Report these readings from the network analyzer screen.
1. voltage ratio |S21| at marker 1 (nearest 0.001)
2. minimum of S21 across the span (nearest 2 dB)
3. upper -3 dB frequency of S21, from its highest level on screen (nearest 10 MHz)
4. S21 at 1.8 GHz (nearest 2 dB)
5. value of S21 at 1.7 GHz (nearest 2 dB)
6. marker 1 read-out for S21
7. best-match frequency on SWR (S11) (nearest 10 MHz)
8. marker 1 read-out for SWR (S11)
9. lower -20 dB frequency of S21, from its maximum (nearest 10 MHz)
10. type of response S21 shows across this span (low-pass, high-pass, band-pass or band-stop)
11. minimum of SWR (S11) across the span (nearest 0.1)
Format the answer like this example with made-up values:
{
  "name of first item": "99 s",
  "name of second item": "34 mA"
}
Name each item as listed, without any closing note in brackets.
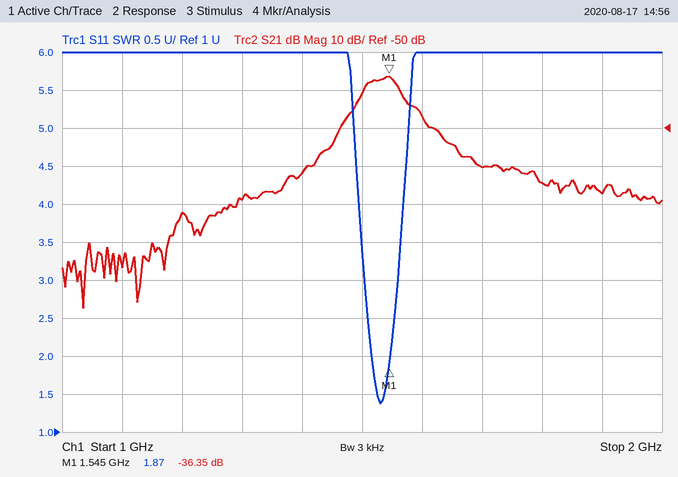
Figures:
{
  "voltage ratio |S21| at marker 1": "0.015",
  "minimum of S21 across the span": "-98 dB",
  "upper -3 dB frequency of S21, from its highest level on screen": "1.56 GHz",
  "S21 at 1.8 GHz": "-64 dB",
  "value of S21 at 1.7 GHz": "-60 dB",
  "marker 1 read-out for S21": "-36.35 dB",
  "best-match frequency on SWR (S11)": "1.53 GHz",
  "marker 1 read-out for SWR": "1.87",
  "lower -20 dB frequency of S21, from its maximum": "1.43 GHz",
  "type of response S21 shows across this span": "band-pass",
  "minimum of SWR (S11) across the span": "1.4"
}
